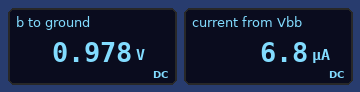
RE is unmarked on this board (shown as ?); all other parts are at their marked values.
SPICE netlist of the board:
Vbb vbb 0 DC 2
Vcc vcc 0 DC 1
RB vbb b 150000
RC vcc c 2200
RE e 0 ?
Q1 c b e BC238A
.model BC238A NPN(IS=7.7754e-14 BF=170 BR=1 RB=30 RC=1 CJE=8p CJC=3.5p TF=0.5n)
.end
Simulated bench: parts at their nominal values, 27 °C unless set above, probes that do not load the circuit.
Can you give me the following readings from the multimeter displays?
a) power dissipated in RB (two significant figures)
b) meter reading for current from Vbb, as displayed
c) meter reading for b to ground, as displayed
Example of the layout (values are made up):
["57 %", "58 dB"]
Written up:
["7.0 µW", "6.8 µA", "0.978 V"]
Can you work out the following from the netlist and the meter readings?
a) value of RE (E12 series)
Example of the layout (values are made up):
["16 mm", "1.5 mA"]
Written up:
["1.8 kΩ"]
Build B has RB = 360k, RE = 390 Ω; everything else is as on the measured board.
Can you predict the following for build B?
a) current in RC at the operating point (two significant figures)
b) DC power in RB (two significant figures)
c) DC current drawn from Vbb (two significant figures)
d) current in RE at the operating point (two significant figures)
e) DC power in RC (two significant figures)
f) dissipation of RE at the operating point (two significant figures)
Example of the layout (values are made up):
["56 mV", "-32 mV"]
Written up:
["330 µA", "4.7 µW", "3.6 µA", "340 µA", "240 µW", "44 µW"]
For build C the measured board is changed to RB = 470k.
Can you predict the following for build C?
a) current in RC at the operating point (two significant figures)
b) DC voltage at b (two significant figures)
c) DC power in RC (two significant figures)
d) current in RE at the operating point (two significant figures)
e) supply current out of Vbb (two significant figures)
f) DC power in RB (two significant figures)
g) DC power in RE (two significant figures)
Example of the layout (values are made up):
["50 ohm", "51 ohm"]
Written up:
["210 µA", "950 mV", "100 µW", "220 µA", "2.2 µA", "2.3 µW", "84 µW"]
